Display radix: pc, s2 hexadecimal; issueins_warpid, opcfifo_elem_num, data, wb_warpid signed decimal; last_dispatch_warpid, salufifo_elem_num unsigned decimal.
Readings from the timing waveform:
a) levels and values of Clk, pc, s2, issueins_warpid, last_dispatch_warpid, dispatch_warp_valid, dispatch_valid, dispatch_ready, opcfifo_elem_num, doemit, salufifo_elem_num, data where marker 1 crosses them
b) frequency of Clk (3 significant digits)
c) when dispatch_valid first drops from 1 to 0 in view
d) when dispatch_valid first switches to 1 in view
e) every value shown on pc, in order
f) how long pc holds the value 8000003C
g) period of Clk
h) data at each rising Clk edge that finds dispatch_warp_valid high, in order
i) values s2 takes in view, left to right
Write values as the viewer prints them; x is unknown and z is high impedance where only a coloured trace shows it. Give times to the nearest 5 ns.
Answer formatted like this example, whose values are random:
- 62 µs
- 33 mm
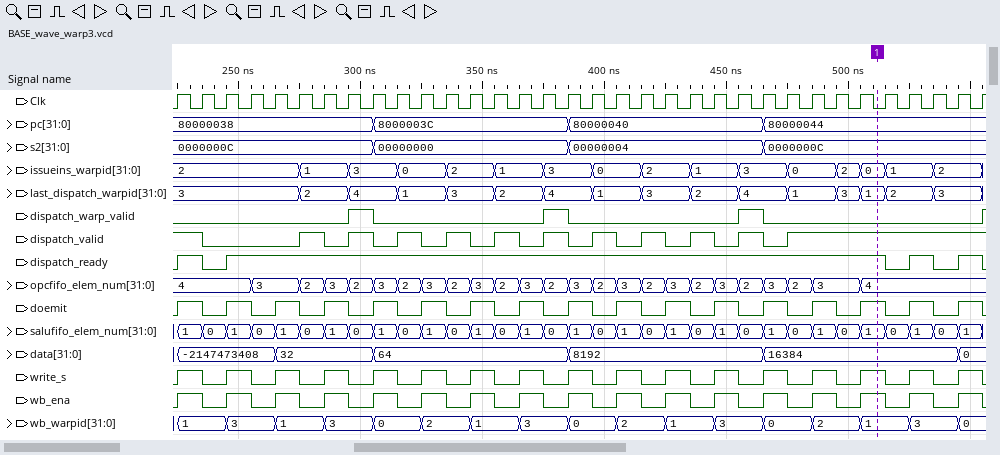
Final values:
- Clk=0, pc=80000044, s2=0000000C, issueins_warpid=0, last_dispatch_warpid=1, dispatch_warp_valid=0, dispatch_valid=1, dispatch_ready=1, opcfifo_elem_num=4, doemit=1, salufifo_elem_num=1, data=16384
- 100 MHz
- 235 ns
- 275 ns
- 80000038, 8000003C, 80000040, 80000044
- 80 ns
- 10 ns
- 32, 64, 8192
- 0000000C, 00000000, 00000004, 0000000C
